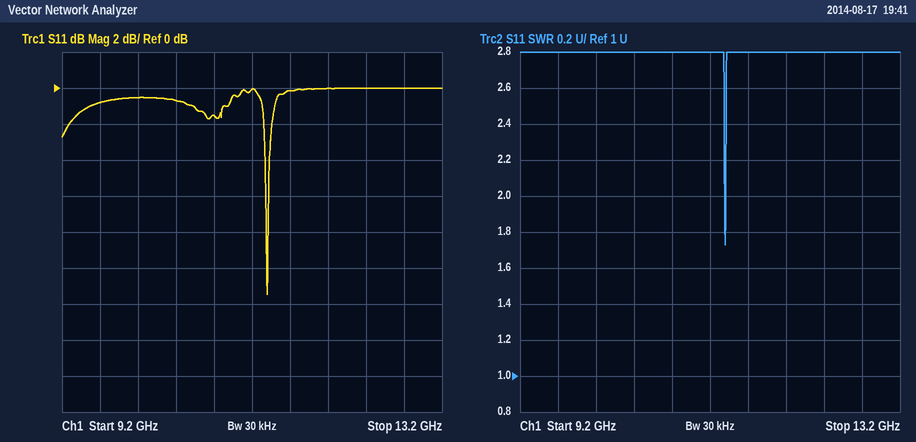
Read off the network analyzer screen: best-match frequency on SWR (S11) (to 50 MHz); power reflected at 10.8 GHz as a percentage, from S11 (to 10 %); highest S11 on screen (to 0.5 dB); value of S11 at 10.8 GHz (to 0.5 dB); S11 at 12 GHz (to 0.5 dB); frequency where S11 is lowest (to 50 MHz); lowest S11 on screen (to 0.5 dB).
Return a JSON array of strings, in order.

["11.35 GHz", "70 %", "0.0 dB", "-1.5 dB", "0.0 dB", "11.35 GHz", "-11.5 dB"]
